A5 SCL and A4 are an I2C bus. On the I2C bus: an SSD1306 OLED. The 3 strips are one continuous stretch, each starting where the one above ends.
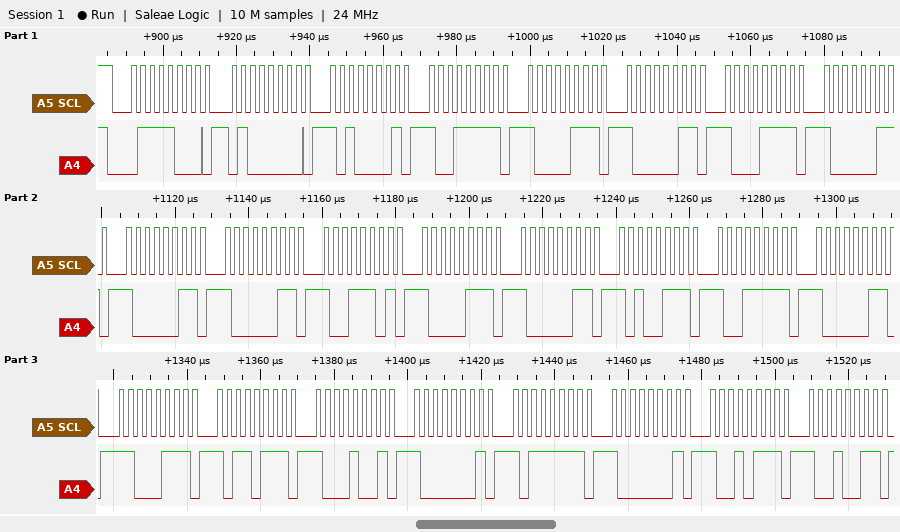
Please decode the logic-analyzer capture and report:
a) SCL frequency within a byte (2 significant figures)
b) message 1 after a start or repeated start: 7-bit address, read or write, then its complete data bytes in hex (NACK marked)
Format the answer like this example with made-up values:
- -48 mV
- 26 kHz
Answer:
- 400 kHz
- 0x3C write: 40 A1 9F 87 83 8F 83 83 83 9D 87 83 A7 9F 83 C7 B7 89 81 BF 81 97 93
